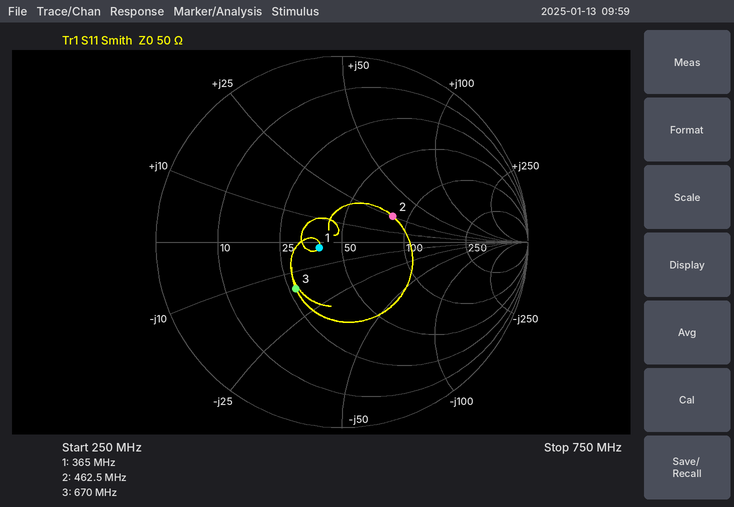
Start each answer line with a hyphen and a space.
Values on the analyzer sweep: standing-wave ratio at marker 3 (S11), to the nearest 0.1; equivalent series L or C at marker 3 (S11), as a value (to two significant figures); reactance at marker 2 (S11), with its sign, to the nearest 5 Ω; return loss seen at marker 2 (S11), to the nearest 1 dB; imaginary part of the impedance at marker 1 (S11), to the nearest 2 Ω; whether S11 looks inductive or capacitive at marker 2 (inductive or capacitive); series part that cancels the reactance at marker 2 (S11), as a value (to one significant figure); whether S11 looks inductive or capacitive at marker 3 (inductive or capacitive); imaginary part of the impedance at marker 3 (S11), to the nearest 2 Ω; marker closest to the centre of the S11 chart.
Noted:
- 2.1
- 15 pF
- +25 Ω
- 10 dB
- -2 Ω
- inductive
- 10 pF
- capacitive
- -16 Ω
- marker 1
